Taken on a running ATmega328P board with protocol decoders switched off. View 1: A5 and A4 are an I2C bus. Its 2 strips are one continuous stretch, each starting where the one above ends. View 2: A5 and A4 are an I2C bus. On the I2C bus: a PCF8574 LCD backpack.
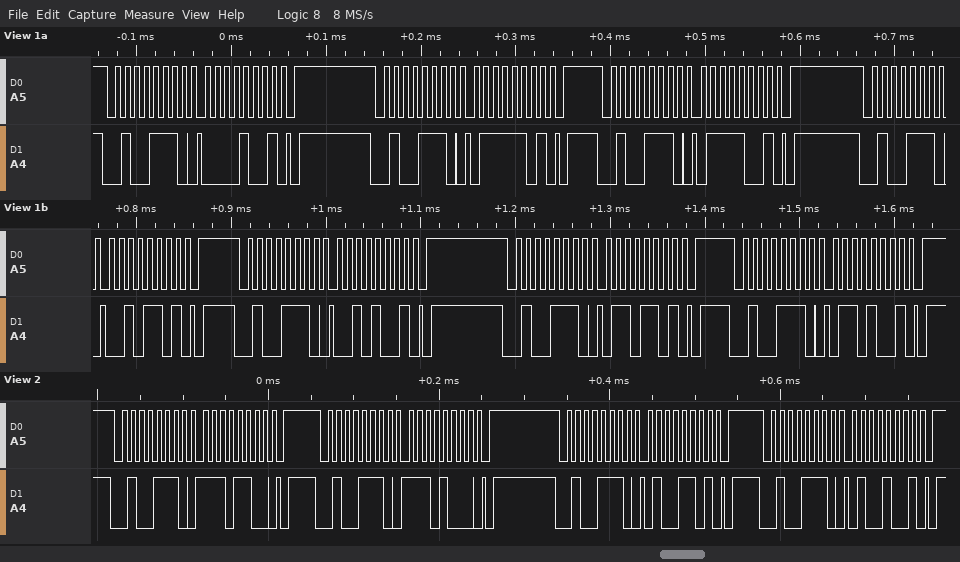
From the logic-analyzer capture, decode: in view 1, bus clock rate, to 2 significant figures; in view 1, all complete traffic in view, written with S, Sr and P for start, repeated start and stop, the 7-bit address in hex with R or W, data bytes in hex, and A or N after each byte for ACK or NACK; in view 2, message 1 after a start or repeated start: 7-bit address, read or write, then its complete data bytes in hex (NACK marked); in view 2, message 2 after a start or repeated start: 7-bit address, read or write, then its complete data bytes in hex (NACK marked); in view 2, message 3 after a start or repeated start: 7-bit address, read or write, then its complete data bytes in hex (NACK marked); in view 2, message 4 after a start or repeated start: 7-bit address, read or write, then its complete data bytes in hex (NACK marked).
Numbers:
100 kHz
S 27W A 09 A P S 27W A 7D A P S 27W A 79 A P S 27W A 2D A P S 27W A 29 A P S 27W A 6D A P S 27W A 69 A P
0x27 write: EC
0x27 write: E8
0x27 write: 4D
0x27 write: 49
